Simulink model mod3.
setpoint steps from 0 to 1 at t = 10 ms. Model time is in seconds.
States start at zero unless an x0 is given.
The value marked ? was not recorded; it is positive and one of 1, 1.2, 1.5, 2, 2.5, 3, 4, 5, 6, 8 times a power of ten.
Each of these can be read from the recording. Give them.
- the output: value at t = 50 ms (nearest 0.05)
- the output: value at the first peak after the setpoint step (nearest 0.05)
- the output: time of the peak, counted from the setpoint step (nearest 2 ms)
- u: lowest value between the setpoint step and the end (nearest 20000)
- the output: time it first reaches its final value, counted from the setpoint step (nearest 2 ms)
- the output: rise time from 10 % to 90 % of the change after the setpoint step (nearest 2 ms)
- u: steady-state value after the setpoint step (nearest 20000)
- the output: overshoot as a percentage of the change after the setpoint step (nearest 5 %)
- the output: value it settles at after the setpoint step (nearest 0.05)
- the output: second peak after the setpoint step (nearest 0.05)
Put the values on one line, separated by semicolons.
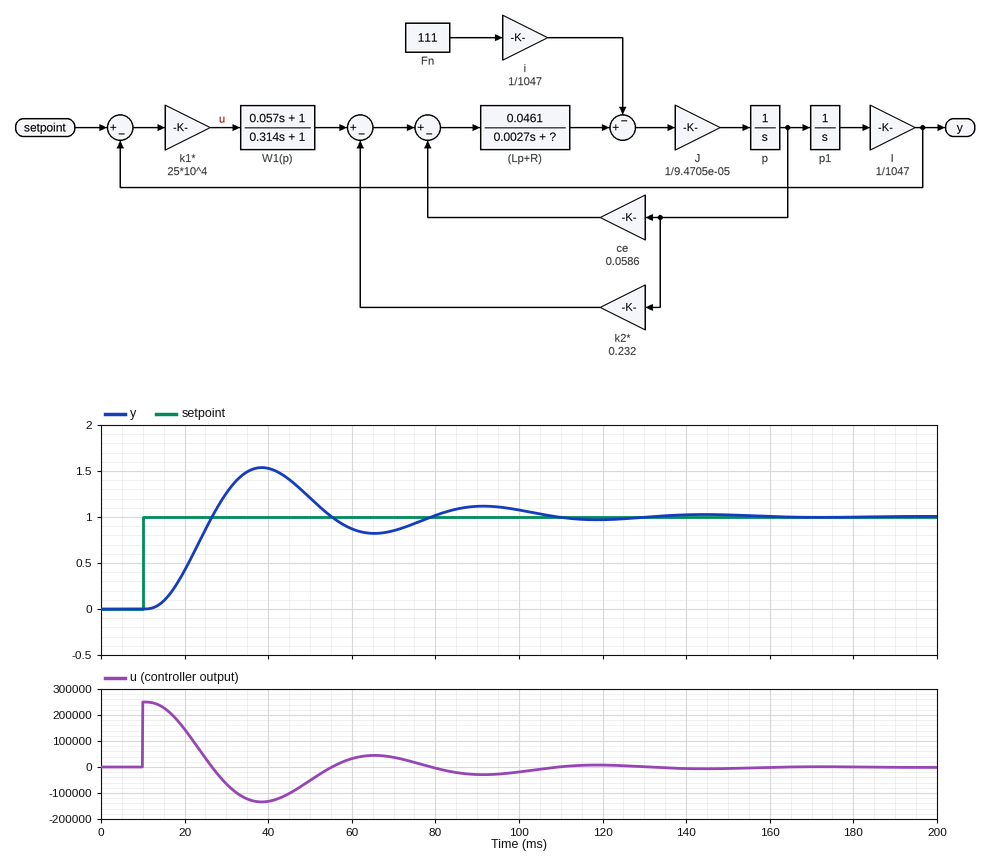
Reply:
1.20; 1.55; 28 ms; -140000; 16 ms; 10 ms; 0; 55 %; 1.00; 1.10
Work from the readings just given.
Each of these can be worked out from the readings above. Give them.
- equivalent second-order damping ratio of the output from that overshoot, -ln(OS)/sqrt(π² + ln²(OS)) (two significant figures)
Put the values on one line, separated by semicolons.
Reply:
0.19
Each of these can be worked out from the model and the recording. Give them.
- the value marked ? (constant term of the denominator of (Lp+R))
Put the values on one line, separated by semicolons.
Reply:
1.5
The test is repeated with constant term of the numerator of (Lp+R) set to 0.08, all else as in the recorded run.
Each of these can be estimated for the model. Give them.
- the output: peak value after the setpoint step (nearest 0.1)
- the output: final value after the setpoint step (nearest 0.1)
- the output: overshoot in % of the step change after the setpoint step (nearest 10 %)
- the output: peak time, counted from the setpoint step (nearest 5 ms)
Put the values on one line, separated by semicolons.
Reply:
1.4; 1.0; 40 %; 20 ms
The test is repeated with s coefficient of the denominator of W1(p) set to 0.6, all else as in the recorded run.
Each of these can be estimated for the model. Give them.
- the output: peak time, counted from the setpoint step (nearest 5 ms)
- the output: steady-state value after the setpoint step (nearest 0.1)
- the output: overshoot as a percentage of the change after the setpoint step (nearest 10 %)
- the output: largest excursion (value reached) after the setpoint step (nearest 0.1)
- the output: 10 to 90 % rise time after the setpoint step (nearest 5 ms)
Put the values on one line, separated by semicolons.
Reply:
40 ms; 1.0; 40 %; 1.4; 15 ms
